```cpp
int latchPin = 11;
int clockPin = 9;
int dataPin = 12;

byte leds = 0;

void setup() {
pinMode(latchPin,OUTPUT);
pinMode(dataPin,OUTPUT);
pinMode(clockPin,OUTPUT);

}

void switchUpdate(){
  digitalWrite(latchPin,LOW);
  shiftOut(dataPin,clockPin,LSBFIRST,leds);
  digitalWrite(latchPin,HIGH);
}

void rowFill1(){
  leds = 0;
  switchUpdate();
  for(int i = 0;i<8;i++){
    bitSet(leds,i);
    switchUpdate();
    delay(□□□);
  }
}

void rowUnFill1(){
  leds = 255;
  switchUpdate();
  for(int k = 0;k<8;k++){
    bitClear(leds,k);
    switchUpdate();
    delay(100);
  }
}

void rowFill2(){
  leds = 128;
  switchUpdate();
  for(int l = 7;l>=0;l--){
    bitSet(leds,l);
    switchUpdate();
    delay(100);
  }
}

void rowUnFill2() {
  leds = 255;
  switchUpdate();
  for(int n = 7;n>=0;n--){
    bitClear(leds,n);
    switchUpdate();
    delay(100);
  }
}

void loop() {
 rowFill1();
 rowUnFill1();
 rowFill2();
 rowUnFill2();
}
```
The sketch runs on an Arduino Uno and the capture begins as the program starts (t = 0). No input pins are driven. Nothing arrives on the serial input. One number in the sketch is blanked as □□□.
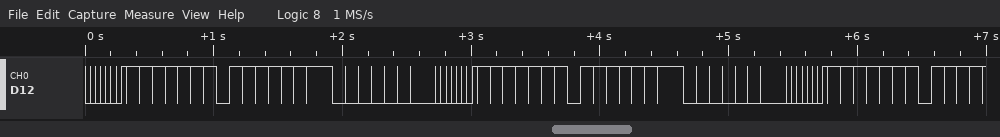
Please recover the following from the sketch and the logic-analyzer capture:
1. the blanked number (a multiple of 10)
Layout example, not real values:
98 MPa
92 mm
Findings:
40
